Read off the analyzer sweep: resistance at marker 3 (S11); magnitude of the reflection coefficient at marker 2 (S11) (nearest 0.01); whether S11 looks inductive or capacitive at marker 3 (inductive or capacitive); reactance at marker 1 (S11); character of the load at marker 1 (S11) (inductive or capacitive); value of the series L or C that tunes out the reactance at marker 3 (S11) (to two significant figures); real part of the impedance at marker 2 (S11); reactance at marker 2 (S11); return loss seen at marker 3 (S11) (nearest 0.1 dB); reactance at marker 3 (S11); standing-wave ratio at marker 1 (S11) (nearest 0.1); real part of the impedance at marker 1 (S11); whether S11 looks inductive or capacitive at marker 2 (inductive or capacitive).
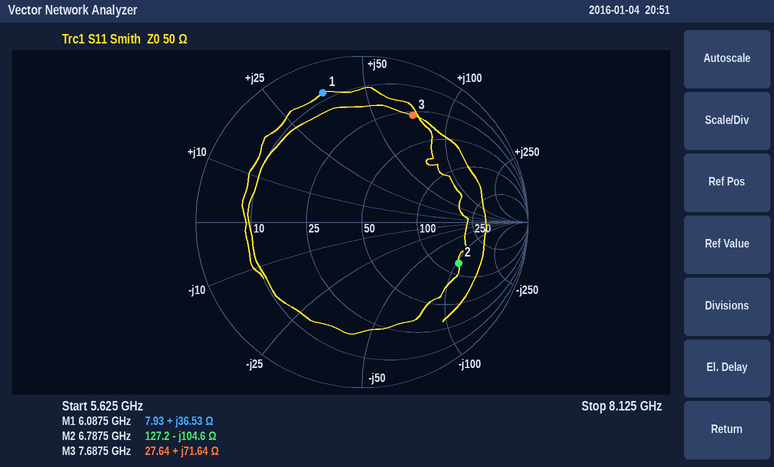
27.64 Ω
0.63
inductive
+36.53 Ω
inductive
290 fF
127.2 Ω
-104.6 Ω
3.0 dB
+71.64 Ω
9.7
7.93 Ω
capacitive
